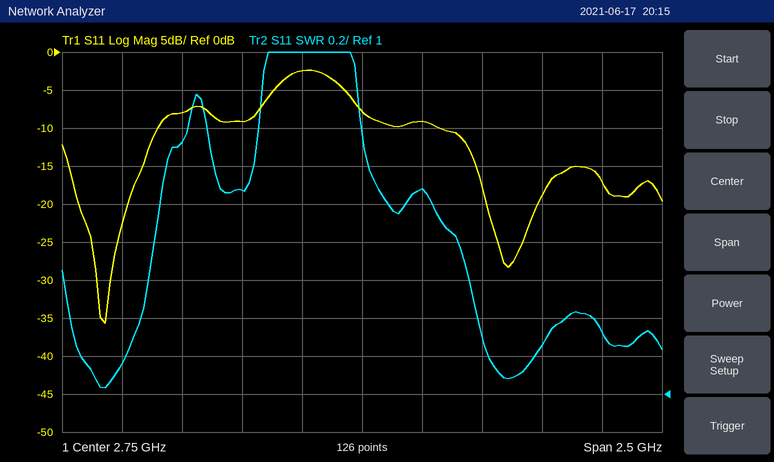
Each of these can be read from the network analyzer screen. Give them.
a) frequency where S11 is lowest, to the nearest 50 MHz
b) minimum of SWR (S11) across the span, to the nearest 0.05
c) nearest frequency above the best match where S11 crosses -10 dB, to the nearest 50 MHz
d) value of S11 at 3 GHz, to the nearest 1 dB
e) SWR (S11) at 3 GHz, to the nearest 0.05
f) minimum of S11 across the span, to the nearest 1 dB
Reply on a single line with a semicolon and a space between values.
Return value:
1.70 GHz; 1.05; 1.90 GHz; -9 dB; 2.10; -36 dB
